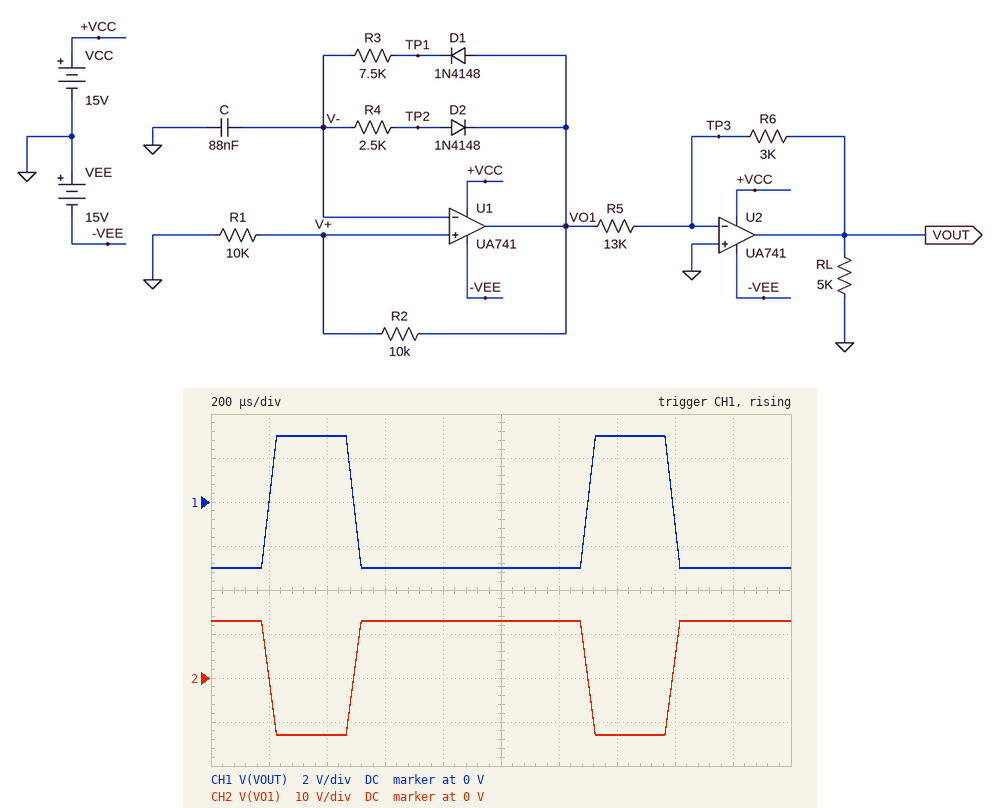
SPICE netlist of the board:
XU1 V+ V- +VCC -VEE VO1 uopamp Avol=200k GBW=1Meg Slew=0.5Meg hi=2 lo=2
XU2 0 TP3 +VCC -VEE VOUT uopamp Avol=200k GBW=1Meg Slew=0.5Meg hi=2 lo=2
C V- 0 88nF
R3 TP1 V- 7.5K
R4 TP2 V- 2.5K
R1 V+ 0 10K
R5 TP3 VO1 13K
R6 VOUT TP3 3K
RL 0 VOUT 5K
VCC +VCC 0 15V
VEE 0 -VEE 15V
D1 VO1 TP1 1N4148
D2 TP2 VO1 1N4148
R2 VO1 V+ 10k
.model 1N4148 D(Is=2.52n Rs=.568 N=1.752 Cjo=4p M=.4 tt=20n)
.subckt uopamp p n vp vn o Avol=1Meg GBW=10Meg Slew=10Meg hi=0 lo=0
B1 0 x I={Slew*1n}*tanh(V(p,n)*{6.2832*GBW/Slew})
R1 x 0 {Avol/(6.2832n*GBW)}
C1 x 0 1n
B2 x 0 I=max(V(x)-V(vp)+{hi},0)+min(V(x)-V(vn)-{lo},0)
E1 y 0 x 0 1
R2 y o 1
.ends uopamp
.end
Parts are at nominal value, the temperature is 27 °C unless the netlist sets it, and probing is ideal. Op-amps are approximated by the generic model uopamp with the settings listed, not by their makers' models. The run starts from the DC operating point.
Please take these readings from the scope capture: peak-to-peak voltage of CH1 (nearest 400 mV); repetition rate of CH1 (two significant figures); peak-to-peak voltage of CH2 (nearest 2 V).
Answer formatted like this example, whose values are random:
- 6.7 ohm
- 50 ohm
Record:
- 6.0 V
- 910 Hz
- 26 V
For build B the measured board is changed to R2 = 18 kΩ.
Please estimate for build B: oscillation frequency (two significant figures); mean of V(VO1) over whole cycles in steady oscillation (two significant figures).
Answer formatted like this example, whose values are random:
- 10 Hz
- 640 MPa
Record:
- 1.3 kHz
- 5.9 V
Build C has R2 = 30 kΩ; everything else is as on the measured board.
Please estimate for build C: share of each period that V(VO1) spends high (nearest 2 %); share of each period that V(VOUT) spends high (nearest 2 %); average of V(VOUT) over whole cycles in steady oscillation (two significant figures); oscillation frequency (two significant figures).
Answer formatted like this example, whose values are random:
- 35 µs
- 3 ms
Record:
- 72 %
- 28 %
- -1.3 V
- 1.8 kHz
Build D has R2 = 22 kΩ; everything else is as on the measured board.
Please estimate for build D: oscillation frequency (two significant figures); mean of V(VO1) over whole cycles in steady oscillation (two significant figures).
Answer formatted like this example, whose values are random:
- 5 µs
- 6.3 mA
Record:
- 1.5 kHz
- 5.9 V
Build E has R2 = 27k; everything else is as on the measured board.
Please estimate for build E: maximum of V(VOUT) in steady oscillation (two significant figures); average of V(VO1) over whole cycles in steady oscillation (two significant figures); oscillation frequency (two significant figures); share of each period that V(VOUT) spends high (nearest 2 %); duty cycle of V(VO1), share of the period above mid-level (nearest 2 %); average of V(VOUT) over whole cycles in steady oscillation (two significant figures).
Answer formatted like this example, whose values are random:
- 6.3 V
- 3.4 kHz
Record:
- 3.0 V
- 5.8 V
- 1.7 kHz
- 28 %
- 72 %
- -1.3 V
